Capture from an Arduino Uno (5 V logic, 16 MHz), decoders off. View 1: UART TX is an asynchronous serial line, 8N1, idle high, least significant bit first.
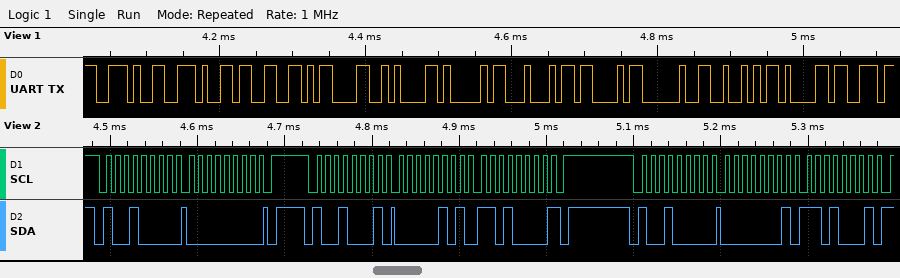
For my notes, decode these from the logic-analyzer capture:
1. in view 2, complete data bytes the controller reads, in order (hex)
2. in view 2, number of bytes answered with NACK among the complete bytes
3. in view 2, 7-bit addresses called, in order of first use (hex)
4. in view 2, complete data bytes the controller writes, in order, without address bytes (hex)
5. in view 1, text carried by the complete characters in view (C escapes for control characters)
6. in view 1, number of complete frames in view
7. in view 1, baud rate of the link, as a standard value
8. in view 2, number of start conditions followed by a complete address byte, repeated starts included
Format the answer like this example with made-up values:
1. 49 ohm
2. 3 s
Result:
1. 05 D0
2. 1
3. 0x48
4. 00 01 D1
5. "..3\r\nADC Ra"
6. 11
7. 115200 baud
8. 3
